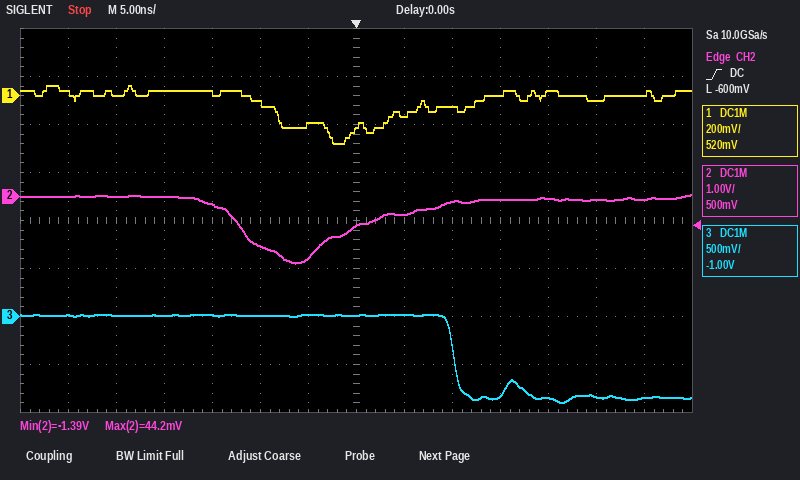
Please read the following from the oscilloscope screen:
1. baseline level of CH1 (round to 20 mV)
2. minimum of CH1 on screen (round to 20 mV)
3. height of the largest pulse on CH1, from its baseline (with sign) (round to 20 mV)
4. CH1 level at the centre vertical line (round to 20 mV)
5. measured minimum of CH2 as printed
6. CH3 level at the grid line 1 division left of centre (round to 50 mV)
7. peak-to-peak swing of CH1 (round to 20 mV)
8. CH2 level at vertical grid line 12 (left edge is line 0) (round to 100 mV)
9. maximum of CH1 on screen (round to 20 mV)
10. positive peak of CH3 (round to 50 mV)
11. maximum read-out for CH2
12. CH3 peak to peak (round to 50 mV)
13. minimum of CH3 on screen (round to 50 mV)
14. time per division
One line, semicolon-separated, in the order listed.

0 mV; -200 mV; -200 mV; -140 mV; -1.39 V; 0 mV; 240 mV; -100 mV; 40 mV; 0 mV; 44.2 mV; 900 mV; -900 mV; 5 ns
